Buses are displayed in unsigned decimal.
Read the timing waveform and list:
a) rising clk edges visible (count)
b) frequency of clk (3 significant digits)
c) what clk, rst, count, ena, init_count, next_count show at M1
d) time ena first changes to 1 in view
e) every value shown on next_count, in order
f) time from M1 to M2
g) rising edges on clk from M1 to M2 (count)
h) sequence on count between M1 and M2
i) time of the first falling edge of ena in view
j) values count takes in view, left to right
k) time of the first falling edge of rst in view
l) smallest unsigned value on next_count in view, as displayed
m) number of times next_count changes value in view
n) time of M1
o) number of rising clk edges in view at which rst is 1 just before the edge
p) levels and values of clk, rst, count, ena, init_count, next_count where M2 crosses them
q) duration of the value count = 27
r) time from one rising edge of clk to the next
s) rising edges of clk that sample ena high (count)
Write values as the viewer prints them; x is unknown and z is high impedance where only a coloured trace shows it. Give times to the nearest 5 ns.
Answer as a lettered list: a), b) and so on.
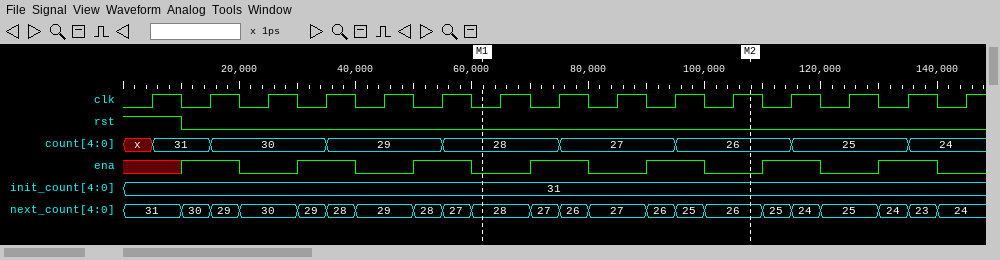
a) 15
b) 100 MHz
c) clk=0, rst=0, count=28, ena=0, init_count=31, next_count=28
d) 10 ns
e) 31, 30, 29, 30, 29, 28, 29, 28, 27, 28, 27, 26, 27, 26, 25, 26, 25, 24, 25, 24, 23, 24
f) 45 ns
g) 5
h) 28, 27, 26
i) 20 ns
j) x, 31, 30, 29, 28, 27, 26, 25, 24
k) 10 ns
l) 23
m) 21
n) 60 ns
o) 1
p) clk=1, rst=0, count=26, ena=0, init_count=31, next_count=26
q) 20 ns
r) 10 ns
s) 7
